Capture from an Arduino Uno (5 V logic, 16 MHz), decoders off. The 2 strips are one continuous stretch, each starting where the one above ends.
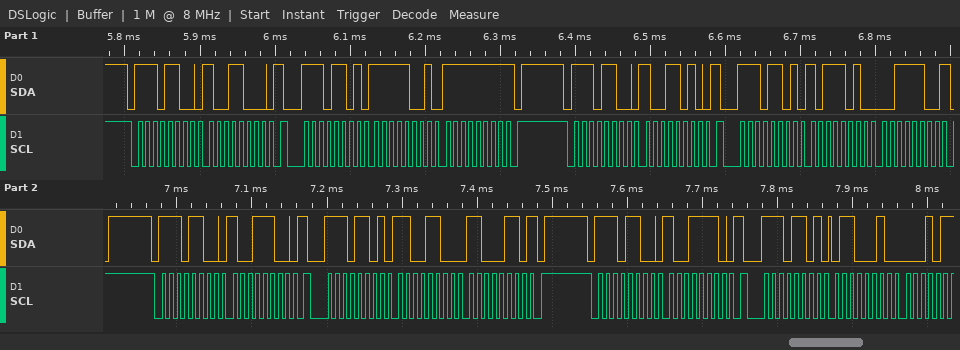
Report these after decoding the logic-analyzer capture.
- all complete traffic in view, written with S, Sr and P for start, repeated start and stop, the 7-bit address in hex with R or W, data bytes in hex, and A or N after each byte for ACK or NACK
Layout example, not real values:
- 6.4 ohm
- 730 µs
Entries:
- S 76W A 98 A Sr 76R A F9 A FF N P S 76W A 9A A Sr 76R A BA A 3C N P S 76W A 9C A Sr 76R A CC A C6 N P S 76W A 9E A Sr 76R A 62 A
